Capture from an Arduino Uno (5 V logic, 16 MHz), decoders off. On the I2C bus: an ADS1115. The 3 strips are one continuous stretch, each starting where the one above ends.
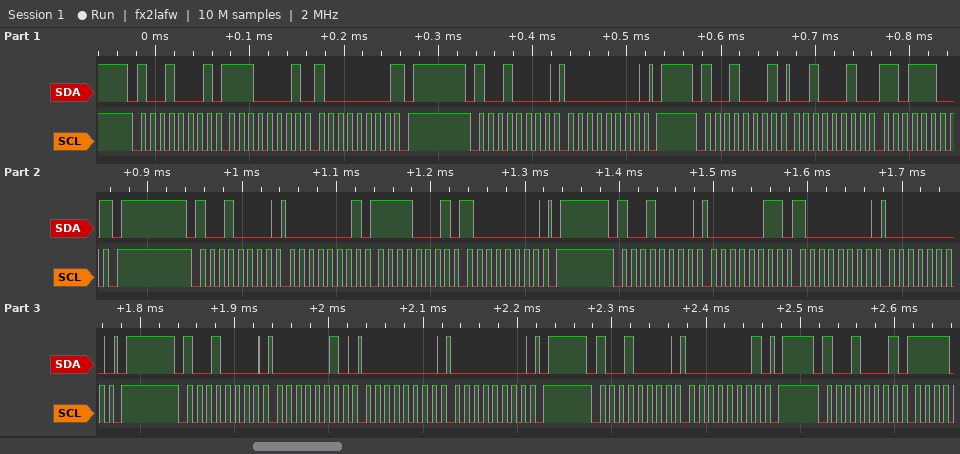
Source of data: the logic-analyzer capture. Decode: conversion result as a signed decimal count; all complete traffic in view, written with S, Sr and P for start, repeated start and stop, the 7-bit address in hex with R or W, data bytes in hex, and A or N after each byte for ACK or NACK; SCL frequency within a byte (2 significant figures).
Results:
8924
S 48R A E1 A 80 N P S 48W A 00 A P S 48R A 22 A DC N P S 48W A 01 A F1 A 80 A P S 48W A 03 A 80 A 00 A P S 48W A 02 A 00 A 00 A P S 48W A 01 A P S 48R A
100 kHz
